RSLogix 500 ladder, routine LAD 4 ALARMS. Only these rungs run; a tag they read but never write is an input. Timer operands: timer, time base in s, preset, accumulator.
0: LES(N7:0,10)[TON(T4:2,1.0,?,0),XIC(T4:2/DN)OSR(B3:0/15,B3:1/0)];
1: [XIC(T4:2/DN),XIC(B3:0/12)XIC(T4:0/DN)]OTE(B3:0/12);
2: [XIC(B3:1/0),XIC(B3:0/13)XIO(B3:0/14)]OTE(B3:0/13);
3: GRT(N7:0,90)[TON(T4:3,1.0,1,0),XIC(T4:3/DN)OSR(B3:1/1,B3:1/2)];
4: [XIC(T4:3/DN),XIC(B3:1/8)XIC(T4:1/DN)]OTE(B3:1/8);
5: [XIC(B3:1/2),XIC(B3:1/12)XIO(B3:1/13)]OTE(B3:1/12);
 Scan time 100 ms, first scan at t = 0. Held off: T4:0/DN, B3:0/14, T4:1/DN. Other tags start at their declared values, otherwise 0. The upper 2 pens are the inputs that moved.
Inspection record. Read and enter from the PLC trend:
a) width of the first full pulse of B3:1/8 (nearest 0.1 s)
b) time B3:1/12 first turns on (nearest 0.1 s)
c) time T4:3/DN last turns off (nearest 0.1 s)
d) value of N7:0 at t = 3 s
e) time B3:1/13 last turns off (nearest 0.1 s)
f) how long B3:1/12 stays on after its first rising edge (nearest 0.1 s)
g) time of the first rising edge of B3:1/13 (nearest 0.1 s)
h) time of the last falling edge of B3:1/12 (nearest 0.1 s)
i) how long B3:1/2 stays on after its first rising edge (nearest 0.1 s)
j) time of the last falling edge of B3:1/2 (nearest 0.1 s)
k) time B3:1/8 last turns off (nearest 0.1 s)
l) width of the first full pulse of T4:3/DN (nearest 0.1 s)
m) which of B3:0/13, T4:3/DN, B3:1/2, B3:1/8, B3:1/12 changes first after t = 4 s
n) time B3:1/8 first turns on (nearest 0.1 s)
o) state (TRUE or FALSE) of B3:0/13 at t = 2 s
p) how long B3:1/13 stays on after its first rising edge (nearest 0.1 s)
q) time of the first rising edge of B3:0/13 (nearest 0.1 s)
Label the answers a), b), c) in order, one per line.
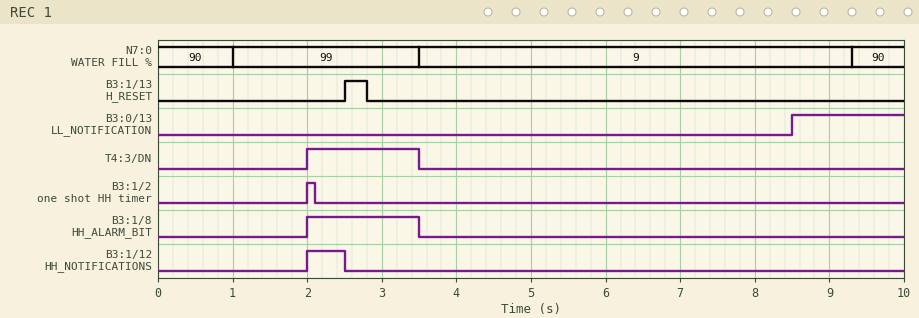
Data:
a) 1.5 s
b) 2.0 s
c) 3.5 s
d) 99
e) 2.8 s
f) 0.5 s
g) 2.5 s
h) 2.5 s
i) 0.1 s
j) 2.1 s
k) 3.5 s
l) 1.5 s
m) B3:0/13
n) 2.0 s
o) FALSE
p) 0.3 s
q) 8.5 s
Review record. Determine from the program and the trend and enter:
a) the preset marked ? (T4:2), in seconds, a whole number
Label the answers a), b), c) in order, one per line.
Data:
a) 5 s
